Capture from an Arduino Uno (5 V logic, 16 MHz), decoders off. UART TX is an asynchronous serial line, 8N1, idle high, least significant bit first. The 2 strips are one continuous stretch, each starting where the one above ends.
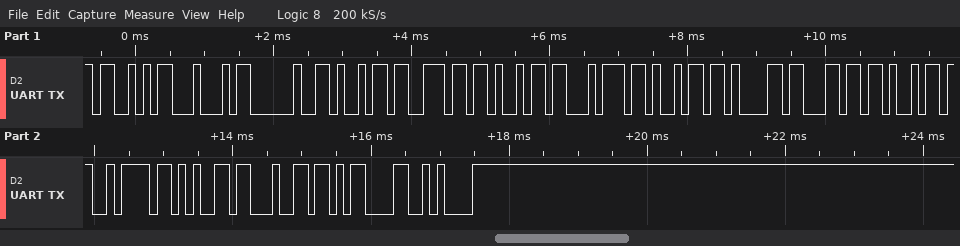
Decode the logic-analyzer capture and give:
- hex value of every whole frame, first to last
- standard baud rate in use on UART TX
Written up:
0x53 0x44 0x20 0x69 0x6E 0x69 0x74 0x69 0x61 0x6C 0x69 0x7A 0x65 0x64 0x0D 0x0A
9600 baud
